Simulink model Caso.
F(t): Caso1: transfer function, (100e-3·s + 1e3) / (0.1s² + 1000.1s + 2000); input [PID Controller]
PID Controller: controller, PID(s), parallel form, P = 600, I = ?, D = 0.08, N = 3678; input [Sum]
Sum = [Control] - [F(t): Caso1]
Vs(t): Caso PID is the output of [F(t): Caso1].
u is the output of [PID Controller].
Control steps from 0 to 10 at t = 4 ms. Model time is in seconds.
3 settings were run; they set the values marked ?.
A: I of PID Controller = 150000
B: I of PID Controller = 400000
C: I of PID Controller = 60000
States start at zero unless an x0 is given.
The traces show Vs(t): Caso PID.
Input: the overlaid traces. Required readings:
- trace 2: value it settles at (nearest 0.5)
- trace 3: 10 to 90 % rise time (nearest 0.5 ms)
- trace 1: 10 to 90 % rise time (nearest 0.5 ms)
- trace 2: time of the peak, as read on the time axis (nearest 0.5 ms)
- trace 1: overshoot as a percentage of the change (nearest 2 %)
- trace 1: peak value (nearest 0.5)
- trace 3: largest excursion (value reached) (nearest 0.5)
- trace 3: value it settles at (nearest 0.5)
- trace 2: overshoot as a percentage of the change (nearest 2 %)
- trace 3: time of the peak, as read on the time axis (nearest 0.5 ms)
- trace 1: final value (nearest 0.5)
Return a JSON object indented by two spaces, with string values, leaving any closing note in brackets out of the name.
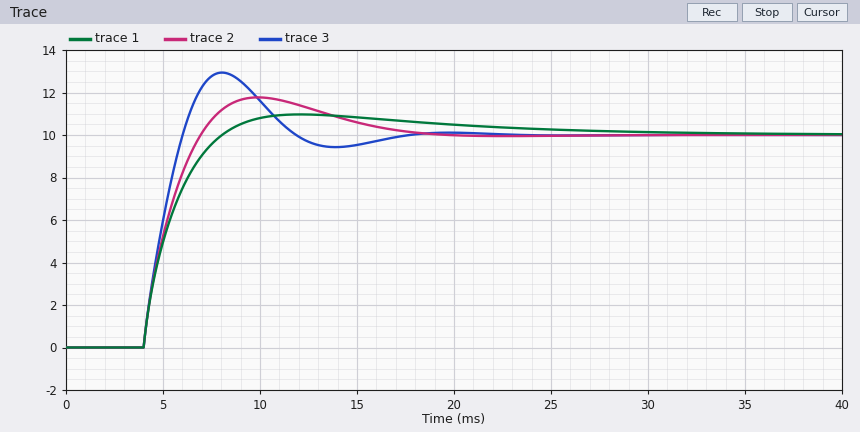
{
  "trace 2: value it settles at": "10.0",
  "trace 3: 10 to 90 % rise time": "1.5 ms",
  "trace 1: 10 to 90 % rise time": "3.0 ms",
  "trace 2: time of the peak, as read on the time axis": "10.0 ms",
  "trace 1: overshoot as a percentage of the change": "10 %",
  "trace 1: peak value": "11.0",
  "trace 3: largest excursion (value reached)": "13.0",
  "trace 3: value it settles at": "10.0",
  "trace 2: overshoot as a percentage of the change": "18 %",
  "trace 3: time of the peak, as read on the time axis": "8.0 ms",
  "trace 1: final value": "10.0"
}
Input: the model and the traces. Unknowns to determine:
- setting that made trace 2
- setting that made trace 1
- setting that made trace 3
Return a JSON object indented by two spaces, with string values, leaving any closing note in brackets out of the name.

{
  "setting that made trace 2": "A",
  "setting that made trace 1": "C",
  "setting that made trace 3": "B"
}
